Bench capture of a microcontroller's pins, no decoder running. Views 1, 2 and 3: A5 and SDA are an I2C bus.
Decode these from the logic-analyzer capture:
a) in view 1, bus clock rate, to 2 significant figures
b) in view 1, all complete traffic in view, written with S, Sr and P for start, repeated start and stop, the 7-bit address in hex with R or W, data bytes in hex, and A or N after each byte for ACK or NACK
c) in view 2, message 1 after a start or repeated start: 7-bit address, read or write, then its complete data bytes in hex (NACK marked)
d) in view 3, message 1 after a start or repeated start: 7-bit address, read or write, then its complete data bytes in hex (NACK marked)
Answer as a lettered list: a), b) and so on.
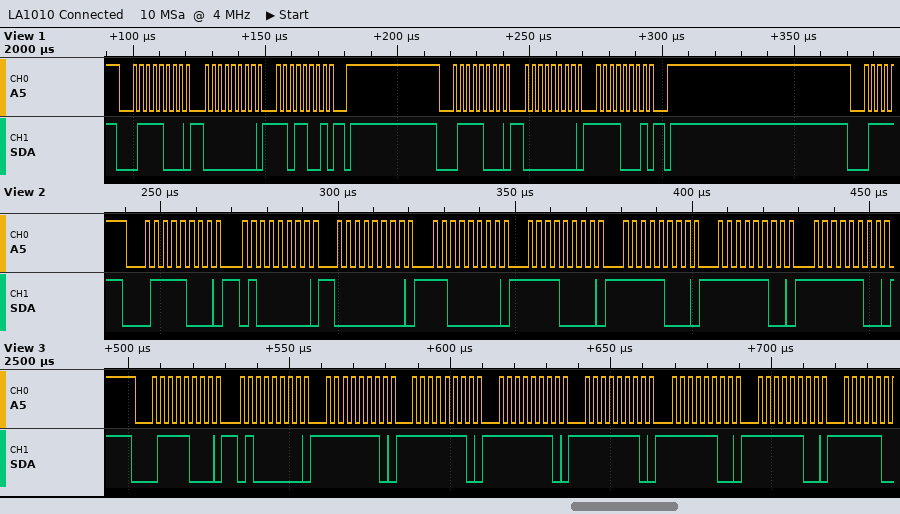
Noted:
a) 400 kHz
b) S 3CW A 00 A D9 A P S 3CW A 00 A F1 A P
c) 0x3C write: 40 00 C0 F0 F8 FC FC
d) 0x3C write: 40 FE FE FE FE FC FC
